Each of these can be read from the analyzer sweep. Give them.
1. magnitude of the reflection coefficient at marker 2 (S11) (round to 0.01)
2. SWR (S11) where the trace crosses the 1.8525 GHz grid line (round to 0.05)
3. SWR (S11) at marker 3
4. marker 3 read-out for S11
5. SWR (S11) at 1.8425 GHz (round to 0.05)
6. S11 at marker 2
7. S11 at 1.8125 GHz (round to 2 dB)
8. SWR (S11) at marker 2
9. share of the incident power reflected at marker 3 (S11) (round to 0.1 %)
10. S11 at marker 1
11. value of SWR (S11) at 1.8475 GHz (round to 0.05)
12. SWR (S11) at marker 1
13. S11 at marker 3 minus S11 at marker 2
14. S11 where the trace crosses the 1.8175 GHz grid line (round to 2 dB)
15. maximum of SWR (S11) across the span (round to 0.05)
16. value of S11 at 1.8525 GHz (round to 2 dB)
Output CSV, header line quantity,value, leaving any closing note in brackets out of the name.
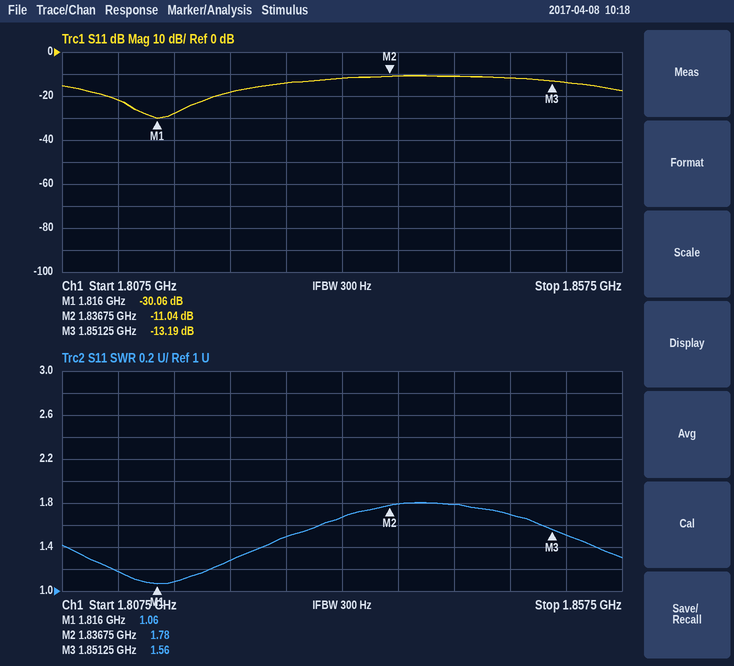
quantity,value
magnitude of the reflection coefficient at marker 2 (S11),0.28
SWR (S11) where the trace crosses the 1.8525 GHz grid line,1.50
SWR (S11) at marker 3,1.56
marker 3 read-out for S11,-13.19 dB
SWR (S11) at 1.8425 GHz,1.80
S11 at marker 2,-11.04 dB
S11 at 1.8125 GHz,-22 dB
SWR (S11) at marker 2,1.78
share of the incident power reflected at marker 3 (S11),4.8 %
S11 at marker 1,-30.06 dB
value of SWR (S11) at 1.8475 GHz,1.70
SWR (S11) at marker 1,1.06
S11 at marker 3 minus S11 at marker 2,-2.15 dB
S11 where the trace crosses the 1.8175 GHz grid line,-28 dB
maximum of SWR (S11) across the span,1.80
value of S11 at 1.8525 GHz,-14 dB
